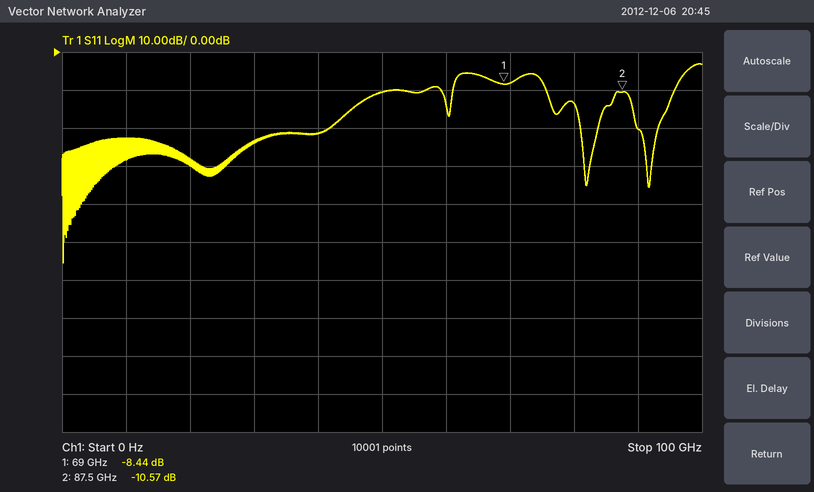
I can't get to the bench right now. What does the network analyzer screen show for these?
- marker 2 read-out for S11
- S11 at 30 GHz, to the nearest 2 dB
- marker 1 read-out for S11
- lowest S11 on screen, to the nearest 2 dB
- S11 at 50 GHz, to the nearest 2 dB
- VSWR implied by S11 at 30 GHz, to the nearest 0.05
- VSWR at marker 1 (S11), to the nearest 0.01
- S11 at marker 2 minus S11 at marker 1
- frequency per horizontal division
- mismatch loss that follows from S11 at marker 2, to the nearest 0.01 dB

-10.57 dB
-24 dB
-8.44 dB
-56 dB
-10 dB
1.15
2.22
-2.13 dB
10 GHz
0.40 dB
